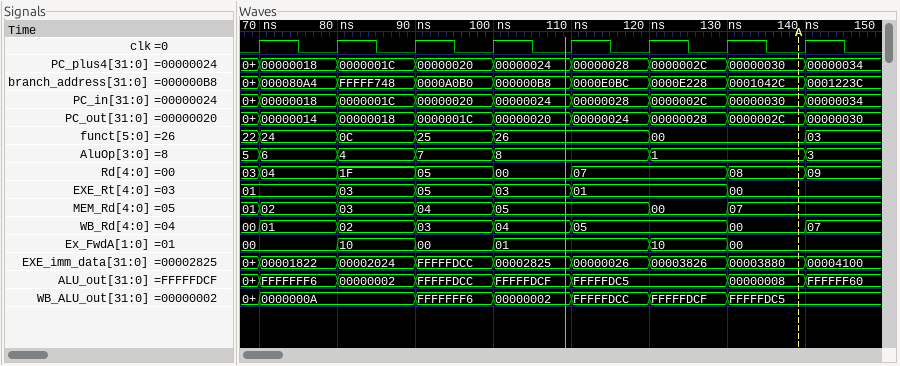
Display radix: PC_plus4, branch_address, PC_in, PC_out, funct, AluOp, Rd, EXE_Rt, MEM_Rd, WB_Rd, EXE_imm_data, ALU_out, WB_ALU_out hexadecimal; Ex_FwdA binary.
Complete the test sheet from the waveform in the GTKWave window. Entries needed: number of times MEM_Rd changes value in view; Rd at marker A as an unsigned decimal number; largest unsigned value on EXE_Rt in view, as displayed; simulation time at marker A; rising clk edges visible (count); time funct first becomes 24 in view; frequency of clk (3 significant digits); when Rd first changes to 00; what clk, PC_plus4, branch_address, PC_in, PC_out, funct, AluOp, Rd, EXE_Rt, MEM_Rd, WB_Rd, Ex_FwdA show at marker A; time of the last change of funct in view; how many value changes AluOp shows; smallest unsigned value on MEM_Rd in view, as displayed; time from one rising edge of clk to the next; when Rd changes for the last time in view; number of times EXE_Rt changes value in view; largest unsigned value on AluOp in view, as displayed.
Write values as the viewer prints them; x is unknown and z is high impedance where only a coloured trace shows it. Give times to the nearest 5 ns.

6
8
05
140 ns
8
70 ns
100 MHz
100 ns
clk=0, PC_plus4=00000030, branch_address=0001042C, PC_in=00000030, PC_out=0000002C, funct=00, AluOp=1, Rd=08, EXE_Rt=00, MEM_Rd=07, WB_Rd=00, Ex_FwdA=00
140 ns
6
00
10 ns
140 ns
5
8
